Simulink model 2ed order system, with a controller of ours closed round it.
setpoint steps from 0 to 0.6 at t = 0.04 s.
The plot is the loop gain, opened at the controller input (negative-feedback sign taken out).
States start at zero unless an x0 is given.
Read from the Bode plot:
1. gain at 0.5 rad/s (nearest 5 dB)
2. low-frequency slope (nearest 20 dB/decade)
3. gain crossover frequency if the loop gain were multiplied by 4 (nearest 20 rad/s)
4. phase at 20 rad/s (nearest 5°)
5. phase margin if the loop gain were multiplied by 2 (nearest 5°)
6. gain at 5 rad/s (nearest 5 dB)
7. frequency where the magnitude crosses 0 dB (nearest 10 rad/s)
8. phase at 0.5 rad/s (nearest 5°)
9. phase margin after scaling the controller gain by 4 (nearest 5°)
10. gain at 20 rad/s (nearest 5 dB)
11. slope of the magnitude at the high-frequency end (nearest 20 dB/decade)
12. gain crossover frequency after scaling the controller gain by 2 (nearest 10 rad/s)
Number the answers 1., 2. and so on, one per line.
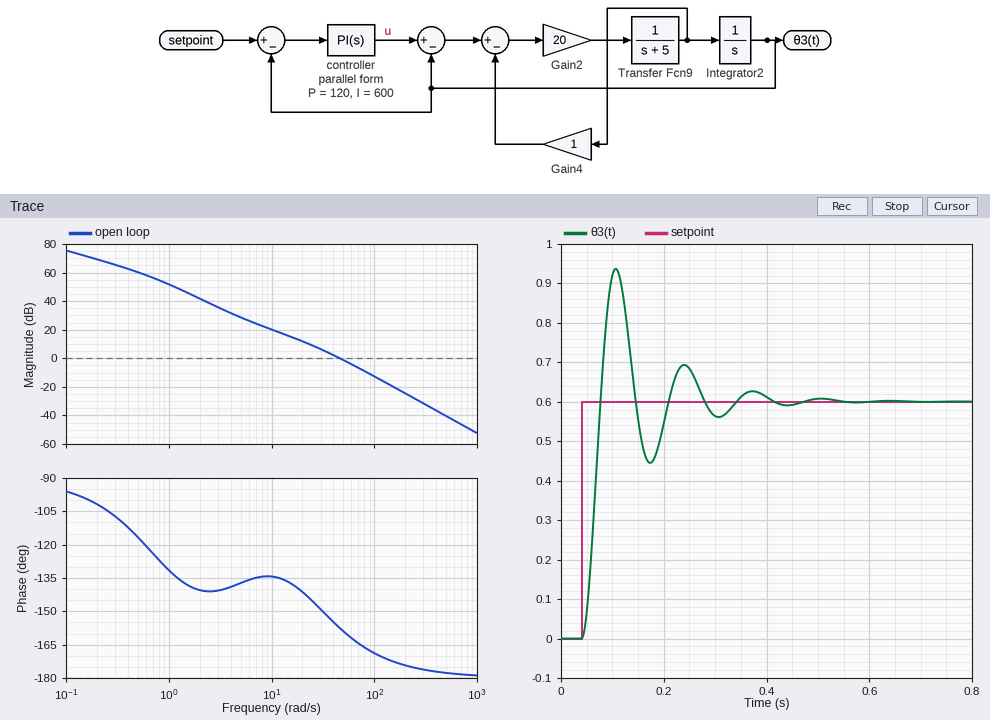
1. 60 dB
2. -20 dB/decade
3. 100 rad/s
4. -140°
5. 15°
6. 30 dB
7. 50 rad/s
8. -115°
9. 10°
10. 10 dB
11. -40 dB/decade
12. 70 rad/s
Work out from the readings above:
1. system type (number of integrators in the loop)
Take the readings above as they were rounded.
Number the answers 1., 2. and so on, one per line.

1. 1
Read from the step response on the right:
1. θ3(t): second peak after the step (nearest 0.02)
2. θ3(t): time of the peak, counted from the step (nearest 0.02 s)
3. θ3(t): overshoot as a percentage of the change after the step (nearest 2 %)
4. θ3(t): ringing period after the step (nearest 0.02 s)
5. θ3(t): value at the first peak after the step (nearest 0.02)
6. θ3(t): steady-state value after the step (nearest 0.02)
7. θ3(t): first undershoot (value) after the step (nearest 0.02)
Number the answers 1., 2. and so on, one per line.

1. 0.70
2. 0.06 s
3. 56 %
4. 0.14 s
5. 0.94
6. 0.60
7. 0.44
